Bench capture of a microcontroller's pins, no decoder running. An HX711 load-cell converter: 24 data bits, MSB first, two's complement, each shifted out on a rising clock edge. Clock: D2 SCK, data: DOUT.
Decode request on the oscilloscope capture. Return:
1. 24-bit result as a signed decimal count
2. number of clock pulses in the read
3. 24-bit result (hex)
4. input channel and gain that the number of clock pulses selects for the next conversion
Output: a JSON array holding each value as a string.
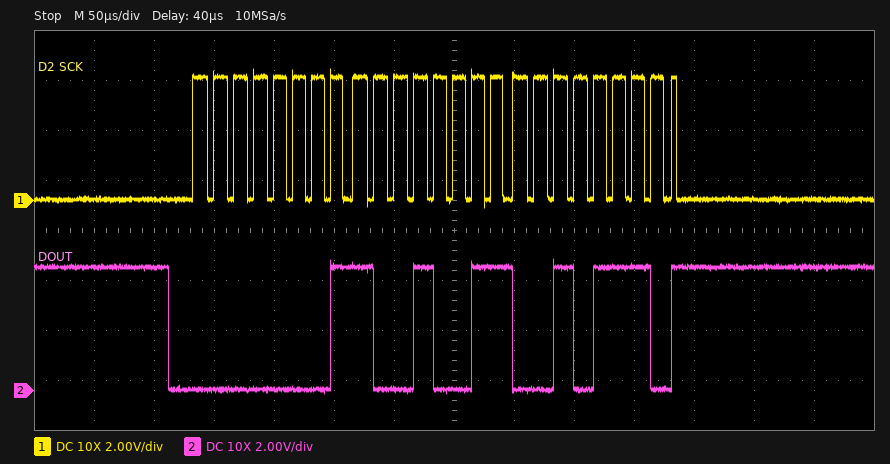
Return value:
["103214", "25", "0x01932E", "channel A, gain 128"]
